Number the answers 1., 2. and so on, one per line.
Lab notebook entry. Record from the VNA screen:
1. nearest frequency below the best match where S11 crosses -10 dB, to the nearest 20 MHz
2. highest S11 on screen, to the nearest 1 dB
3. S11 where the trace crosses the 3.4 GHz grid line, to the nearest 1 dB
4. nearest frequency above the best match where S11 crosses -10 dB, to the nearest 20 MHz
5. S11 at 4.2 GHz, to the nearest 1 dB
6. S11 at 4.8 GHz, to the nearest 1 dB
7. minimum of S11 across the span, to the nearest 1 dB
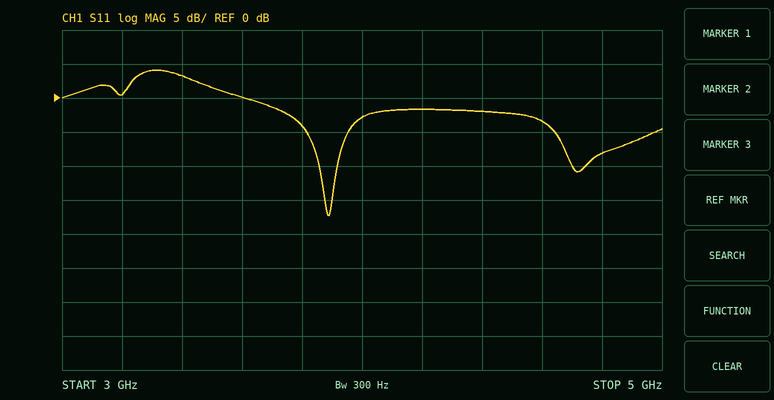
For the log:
1. 3.86 GHz
2. 4 dB
3. 3 dB
4. 3.92 GHz
5. -2 dB
6. -8 dB
7. -17 dB
